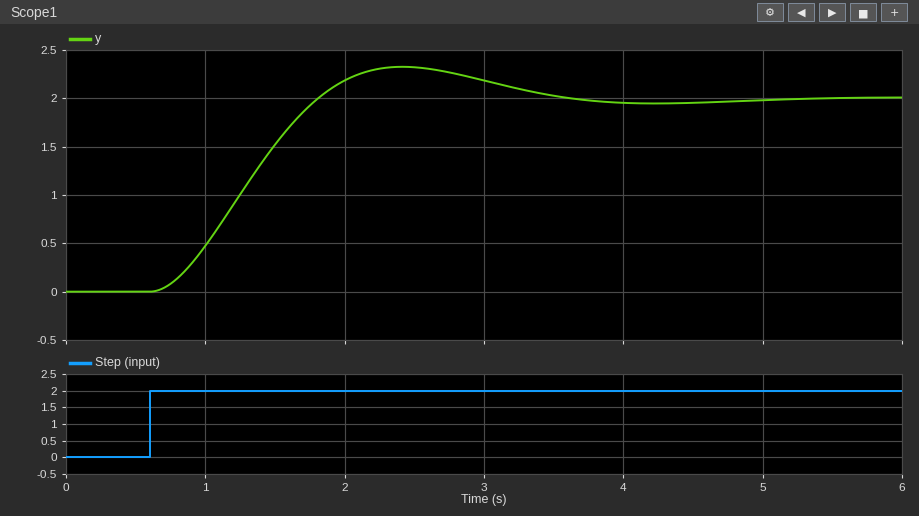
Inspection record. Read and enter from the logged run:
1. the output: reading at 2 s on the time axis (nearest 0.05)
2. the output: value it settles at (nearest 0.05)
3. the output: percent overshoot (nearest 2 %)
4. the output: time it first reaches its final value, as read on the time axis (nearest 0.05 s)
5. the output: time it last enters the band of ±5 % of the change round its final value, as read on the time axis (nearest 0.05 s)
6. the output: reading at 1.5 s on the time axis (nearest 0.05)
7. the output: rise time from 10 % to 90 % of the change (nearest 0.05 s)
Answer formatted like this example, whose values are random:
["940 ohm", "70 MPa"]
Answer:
["2.20", "2.00", "16 %", "1.80 s", "3.25 s", "1.50", "0.80 s"]
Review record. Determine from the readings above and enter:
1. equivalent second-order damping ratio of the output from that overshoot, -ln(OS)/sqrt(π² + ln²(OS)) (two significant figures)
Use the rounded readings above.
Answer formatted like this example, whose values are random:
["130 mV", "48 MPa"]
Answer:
["0.50"]
